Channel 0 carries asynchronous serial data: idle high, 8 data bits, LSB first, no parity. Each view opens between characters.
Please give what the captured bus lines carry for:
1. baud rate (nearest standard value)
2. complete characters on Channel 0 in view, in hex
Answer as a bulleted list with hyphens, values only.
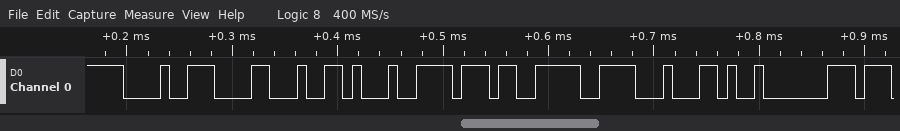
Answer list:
- 115200 baud
- C8, 18, 16, DE, F3, 1E, 2C, C0
